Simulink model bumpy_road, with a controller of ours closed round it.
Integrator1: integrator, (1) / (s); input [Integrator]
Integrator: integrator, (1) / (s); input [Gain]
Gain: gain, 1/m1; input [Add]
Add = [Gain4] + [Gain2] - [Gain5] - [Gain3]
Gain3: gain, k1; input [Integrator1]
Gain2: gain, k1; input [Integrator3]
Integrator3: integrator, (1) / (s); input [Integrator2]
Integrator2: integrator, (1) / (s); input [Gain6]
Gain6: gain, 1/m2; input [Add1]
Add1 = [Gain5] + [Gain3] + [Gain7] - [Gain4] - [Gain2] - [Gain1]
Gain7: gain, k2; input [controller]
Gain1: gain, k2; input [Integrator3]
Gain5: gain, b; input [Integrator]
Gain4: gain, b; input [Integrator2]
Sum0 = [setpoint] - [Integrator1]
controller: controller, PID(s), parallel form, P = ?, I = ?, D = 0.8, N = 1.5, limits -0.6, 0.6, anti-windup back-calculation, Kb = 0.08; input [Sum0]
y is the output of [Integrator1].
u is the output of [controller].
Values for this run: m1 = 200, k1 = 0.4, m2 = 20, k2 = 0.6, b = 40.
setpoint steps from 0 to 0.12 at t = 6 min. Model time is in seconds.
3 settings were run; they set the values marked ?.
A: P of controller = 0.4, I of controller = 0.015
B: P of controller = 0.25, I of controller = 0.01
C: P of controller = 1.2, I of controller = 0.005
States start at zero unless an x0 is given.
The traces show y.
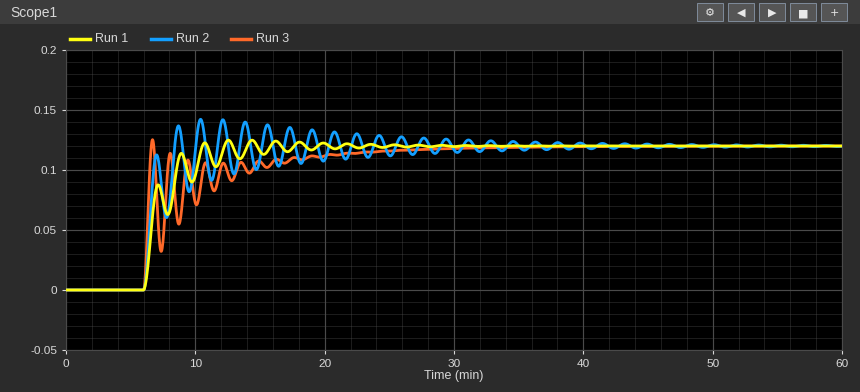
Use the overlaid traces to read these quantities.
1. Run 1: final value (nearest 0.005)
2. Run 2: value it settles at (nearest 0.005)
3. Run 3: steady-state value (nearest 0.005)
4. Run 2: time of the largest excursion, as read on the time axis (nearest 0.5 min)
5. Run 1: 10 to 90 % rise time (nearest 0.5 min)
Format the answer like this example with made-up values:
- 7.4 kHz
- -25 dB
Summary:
- 0.120
- 0.120
- 0.120
- 10.5 min
- 2.5 min
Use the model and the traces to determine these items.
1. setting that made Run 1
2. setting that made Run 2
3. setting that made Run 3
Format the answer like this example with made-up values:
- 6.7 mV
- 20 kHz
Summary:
- B
- A
- C
